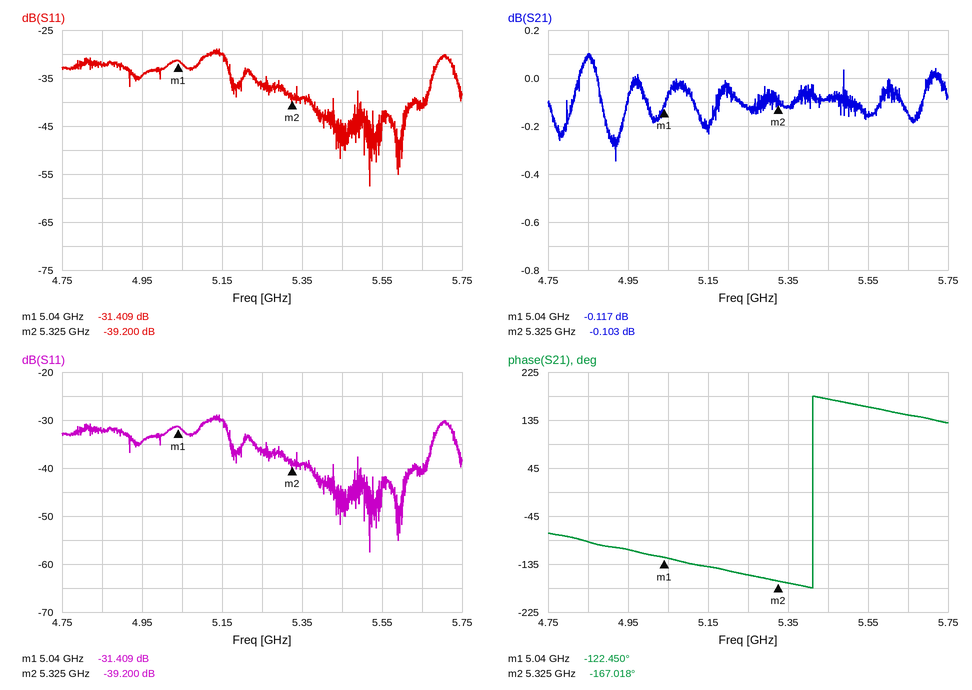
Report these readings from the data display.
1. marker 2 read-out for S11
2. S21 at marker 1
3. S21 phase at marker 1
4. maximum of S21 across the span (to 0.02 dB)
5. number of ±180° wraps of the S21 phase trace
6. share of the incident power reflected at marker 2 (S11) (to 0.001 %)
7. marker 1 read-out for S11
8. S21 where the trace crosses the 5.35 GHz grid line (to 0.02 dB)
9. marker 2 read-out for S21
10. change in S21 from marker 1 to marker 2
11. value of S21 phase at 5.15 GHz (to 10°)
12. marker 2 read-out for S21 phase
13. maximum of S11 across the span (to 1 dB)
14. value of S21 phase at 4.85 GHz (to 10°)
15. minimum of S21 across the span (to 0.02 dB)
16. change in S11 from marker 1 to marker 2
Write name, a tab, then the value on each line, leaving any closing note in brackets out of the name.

marker 2 read-out for S11	-39.200 dB
S21 at marker 1	-0.117 dB
S21 phase at marker 1	-122.450°
maximum of S21 across the span	0.10 dB
number of ±180° wraps of the S21 phase trace	1
share of the incident power reflected at marker 2 (S11)	0.012 %
marker 1 read-out for S11	-31.409 dB
S21 where the trace crosses the 5.35 GHz grid line	-0.12 dB
marker 2 read-out for S21	-0.103 dB
change in S21 from marker 1 to marker 2	0.014 dB
value of S21 phase at 5.15 GHz	-140°
marker 2 read-out for S21 phase	-167.018°
maximum of S11 across the span	-29 dB
value of S21 phase at 4.85 GHz	-90°
minimum of S21 across the span	-0.34 dB
change in S11 from marker 1 to marker 2	-7.791 dB
